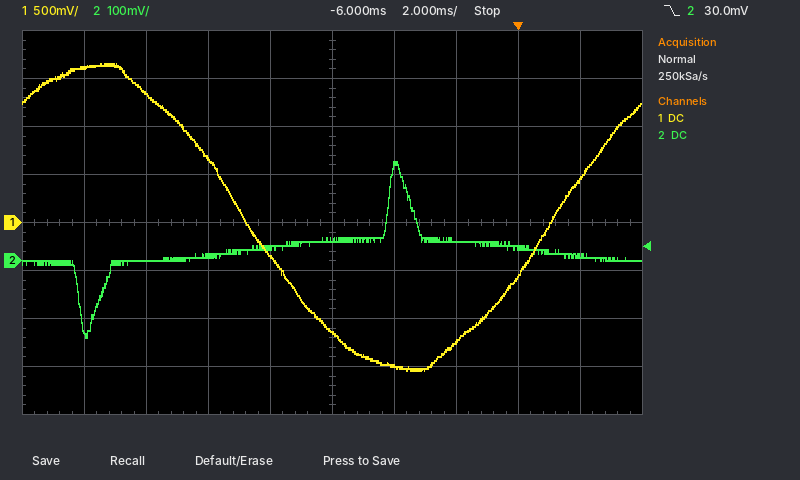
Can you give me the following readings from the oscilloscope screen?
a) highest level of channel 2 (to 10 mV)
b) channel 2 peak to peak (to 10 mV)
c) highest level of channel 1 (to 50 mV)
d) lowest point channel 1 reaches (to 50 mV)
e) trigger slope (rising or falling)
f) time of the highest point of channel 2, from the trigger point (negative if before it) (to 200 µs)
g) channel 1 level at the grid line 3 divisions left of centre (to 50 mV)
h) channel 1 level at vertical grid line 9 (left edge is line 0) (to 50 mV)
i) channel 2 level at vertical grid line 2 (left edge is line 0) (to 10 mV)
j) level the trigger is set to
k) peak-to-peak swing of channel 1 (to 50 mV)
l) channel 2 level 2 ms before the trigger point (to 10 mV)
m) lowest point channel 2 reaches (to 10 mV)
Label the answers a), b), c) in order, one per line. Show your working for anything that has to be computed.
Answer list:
a) 210 mV
b) 210 mV − (-160 mV) = 370 mV
c) 1.65 V
d) -1.55 V
e) falling
f) -4.0 ms
g) 1.35 V
h) 450 mV
i) 0 mV
j) 30.0 mV
k) 1.65 V − (-1.55 V) = 3.20 V
l) 40 mV
m) -160 mV
